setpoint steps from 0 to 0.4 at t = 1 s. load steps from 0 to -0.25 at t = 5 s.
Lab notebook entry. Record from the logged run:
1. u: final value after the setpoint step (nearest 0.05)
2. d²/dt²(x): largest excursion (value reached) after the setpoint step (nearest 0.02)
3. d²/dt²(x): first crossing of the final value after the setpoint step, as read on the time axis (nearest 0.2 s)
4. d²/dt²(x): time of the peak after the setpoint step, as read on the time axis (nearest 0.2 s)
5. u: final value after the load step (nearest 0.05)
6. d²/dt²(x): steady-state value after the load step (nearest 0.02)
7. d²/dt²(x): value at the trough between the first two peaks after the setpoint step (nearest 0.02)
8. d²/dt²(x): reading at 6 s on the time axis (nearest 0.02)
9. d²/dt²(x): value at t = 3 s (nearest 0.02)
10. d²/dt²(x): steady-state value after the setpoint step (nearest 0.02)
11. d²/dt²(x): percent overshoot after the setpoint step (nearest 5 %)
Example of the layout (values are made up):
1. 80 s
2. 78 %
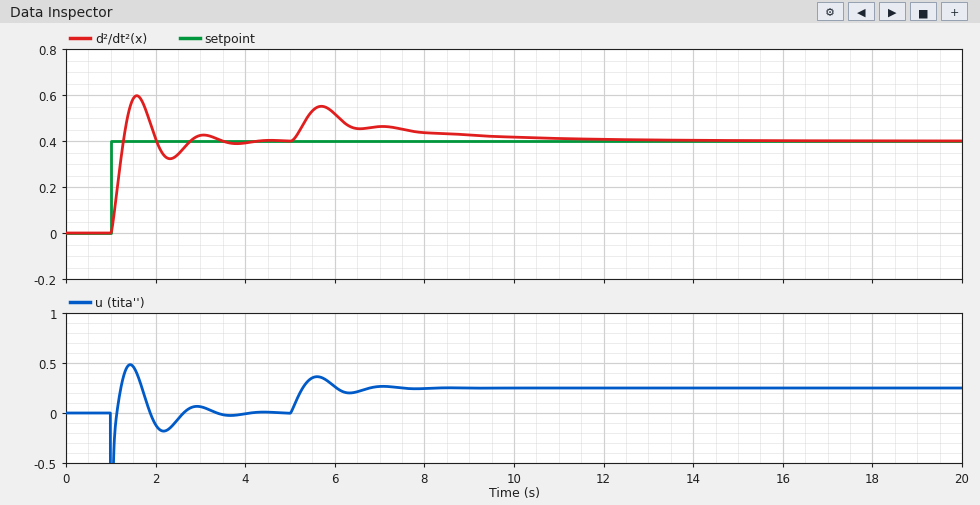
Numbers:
1. 0.00
2. 0.60
3. 1.2 s
4. 1.6 s
5. 0.25
6. 0.40
7. 0.32
8. 0.52
9. 0.42
10. 0.40
11. 50 %
